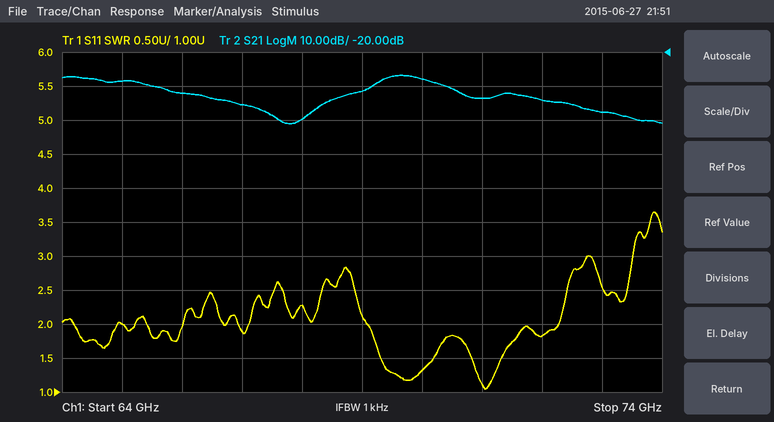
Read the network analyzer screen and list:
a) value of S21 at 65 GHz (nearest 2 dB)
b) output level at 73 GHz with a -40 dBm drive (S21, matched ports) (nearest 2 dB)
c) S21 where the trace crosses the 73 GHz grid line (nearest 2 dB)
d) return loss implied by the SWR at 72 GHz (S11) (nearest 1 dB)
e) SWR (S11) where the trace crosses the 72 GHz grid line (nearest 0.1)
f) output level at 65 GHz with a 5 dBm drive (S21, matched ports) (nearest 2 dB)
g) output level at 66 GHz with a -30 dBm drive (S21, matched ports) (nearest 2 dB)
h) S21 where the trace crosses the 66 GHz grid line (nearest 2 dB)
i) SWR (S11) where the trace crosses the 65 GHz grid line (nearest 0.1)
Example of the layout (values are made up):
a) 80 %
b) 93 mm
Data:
a) -28 dB
b) -78 dBm
c) -38 dB
d) 11 dB
e) 1.8
f) -24 dBm
g) -62 dBm
h) -32 dB
i) 2.0
